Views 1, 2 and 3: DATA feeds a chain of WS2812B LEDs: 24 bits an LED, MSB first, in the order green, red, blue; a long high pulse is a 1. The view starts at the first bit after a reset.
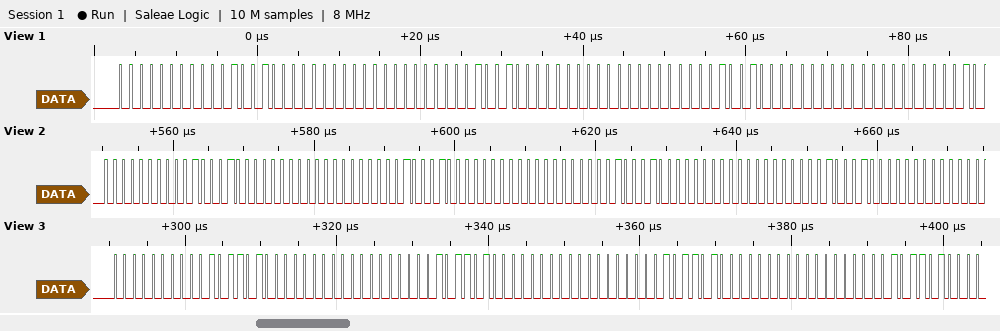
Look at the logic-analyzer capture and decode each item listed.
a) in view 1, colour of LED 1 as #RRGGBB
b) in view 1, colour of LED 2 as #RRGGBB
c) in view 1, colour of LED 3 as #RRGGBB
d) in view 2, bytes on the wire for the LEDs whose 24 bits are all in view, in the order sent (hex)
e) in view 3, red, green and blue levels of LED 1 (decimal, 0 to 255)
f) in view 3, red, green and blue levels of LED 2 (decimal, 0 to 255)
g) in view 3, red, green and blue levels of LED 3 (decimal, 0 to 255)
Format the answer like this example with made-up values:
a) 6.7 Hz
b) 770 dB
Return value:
a) #120000
b) #120000
c) #120000
d) 00 22 00 00 22 00 00 22 00 00 22 00
e) 45, 0, 0
f) 45, 0, 0
g) 45, 0, 0
